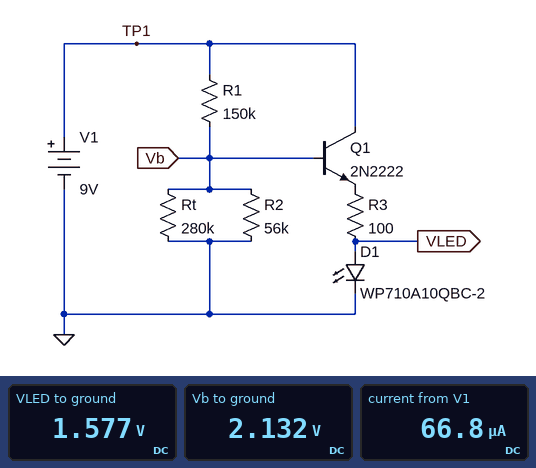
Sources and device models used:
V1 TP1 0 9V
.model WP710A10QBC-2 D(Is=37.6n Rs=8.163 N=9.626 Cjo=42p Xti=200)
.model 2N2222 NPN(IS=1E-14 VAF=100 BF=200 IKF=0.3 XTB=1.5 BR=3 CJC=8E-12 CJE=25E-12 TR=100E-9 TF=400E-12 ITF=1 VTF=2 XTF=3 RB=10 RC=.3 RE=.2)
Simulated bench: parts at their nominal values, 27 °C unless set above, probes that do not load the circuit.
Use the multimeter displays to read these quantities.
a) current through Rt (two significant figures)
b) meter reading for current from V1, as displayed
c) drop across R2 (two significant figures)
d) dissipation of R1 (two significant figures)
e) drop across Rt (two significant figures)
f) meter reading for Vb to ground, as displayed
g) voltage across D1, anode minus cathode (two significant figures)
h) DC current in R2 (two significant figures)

7.6 µA
66.8 µA
2.1 V
310 µW
2.1 V
2.132 V
1.6 V
38 µA
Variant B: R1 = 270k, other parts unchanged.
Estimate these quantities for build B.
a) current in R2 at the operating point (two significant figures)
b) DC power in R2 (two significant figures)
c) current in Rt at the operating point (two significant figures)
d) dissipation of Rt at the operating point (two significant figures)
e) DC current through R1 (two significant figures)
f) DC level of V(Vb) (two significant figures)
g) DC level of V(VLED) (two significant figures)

24 µA
31 µW
4.7 µA
6.3 µW
28 µA
1.3 V
850 mV
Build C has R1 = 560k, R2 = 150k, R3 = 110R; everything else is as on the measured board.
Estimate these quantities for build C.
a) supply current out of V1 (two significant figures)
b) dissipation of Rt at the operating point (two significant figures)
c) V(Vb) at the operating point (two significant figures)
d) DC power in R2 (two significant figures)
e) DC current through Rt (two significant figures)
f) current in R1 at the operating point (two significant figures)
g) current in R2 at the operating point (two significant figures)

15 µA
6.4 µW
1.3 V
12 µW
4.8 µA
14 µA
8.9 µA
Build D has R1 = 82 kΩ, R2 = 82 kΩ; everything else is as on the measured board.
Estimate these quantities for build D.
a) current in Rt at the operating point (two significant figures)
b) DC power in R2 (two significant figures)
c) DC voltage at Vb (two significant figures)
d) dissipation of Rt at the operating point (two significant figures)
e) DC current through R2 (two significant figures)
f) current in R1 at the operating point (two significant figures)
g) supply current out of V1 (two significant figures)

13 µA
160 µW
3.6 V
46 µW
44 µA
66 µA
2.0 mA
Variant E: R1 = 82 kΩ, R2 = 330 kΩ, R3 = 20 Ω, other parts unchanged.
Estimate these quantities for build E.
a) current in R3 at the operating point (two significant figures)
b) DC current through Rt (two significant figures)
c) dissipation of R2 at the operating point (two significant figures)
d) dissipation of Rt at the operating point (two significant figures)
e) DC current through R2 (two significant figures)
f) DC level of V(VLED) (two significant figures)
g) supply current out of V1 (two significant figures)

7.3 mA
14 µA
47 µW
56 µW
12 µA
3.1 V
7.4 mA
